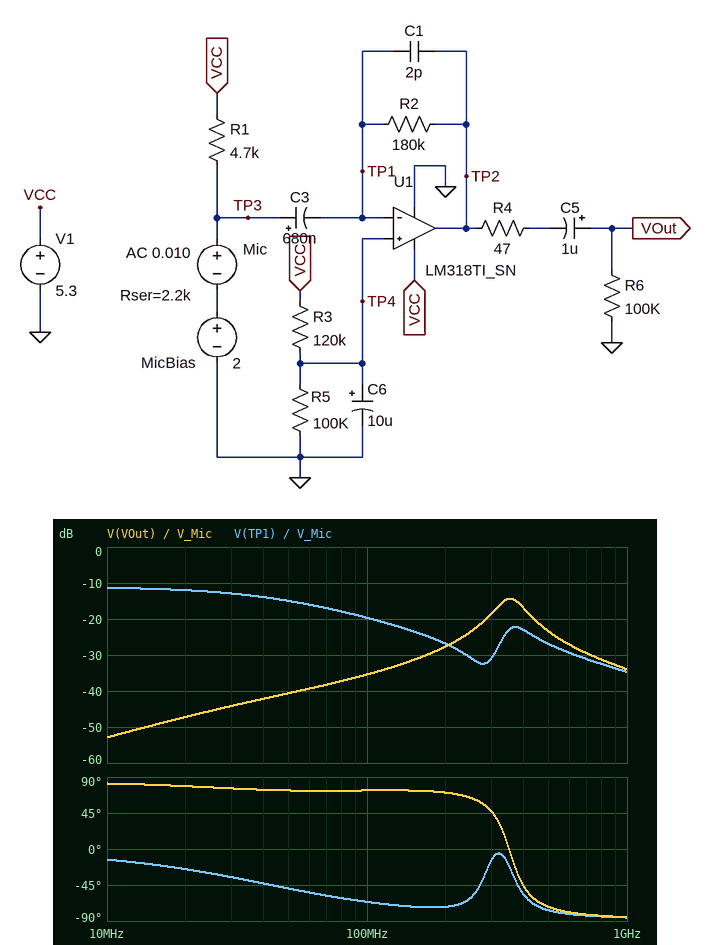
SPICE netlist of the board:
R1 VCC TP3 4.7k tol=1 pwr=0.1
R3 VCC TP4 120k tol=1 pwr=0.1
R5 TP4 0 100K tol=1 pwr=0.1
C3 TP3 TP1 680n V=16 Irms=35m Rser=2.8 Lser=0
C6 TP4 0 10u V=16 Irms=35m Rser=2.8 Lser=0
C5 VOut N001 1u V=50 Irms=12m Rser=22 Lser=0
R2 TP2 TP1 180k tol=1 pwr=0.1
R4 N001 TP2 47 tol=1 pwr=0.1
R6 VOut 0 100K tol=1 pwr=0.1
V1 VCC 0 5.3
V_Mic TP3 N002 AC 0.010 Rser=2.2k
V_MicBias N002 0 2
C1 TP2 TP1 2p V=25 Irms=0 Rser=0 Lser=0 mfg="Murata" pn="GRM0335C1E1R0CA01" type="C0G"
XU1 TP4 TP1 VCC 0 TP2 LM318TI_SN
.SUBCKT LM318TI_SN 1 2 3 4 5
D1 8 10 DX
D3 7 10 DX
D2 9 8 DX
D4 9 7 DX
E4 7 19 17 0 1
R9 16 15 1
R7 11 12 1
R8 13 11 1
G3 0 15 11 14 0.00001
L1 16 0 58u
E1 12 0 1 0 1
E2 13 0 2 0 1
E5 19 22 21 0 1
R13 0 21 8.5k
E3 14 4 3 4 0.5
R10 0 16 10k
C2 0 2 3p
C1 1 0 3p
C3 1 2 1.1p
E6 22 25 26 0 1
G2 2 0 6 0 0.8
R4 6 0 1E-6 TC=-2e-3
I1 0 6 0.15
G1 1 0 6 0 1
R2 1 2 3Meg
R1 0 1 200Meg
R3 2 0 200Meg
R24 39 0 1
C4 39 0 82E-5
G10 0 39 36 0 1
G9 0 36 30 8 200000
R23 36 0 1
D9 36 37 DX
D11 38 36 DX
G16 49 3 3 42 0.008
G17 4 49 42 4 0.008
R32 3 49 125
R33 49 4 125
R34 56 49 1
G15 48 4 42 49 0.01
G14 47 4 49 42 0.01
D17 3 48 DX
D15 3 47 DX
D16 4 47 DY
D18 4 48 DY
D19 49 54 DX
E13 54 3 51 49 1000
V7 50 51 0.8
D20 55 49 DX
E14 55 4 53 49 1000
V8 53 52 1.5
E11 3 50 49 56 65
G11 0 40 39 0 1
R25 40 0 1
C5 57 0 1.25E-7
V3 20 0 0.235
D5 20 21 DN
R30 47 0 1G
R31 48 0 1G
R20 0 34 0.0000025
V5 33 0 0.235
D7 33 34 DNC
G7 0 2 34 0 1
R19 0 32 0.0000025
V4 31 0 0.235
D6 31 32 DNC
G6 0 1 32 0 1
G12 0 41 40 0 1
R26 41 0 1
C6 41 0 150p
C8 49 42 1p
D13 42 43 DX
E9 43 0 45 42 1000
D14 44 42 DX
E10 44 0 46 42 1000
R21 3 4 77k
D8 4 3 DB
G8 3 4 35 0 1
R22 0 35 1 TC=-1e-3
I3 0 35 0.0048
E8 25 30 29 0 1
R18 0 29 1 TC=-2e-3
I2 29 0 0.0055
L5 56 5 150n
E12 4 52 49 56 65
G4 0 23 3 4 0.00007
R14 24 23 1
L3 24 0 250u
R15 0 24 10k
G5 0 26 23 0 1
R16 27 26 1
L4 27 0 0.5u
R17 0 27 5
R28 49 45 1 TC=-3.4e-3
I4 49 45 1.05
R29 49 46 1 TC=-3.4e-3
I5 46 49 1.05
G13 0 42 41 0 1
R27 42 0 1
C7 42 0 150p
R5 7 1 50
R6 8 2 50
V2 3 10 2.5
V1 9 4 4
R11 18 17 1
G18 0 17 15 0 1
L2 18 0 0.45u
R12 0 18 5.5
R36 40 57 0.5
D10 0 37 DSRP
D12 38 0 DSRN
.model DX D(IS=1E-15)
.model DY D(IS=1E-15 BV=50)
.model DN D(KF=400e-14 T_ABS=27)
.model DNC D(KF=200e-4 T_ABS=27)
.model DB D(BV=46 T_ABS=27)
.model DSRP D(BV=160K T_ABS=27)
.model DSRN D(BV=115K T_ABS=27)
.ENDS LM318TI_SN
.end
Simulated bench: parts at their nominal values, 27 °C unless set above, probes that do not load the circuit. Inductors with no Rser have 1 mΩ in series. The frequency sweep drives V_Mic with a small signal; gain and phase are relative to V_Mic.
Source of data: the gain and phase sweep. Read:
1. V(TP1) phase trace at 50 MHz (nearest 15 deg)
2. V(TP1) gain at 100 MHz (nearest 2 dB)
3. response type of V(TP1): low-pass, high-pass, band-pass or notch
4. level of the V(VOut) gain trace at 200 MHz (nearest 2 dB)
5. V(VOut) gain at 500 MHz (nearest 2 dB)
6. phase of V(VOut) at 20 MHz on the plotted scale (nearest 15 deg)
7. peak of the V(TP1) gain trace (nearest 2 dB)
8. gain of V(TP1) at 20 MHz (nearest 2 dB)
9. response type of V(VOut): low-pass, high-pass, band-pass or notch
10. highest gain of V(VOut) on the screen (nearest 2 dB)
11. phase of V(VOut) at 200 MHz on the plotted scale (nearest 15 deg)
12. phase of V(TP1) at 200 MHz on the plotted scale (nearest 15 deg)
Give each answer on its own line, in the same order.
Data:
-45 deg
-20 dB
low-pass
-28 dB
-24 dB
75 deg
-12 dB
-12 dB
band-pass
-14 dB
75 deg
-75 deg
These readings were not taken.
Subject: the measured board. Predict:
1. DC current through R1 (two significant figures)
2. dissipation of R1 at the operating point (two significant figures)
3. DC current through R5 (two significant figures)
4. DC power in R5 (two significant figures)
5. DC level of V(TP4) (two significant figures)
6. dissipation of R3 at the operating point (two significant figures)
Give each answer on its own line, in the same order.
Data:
480 µA
1.1 mW
34 µA
110 µW
3.4 V
31 µW
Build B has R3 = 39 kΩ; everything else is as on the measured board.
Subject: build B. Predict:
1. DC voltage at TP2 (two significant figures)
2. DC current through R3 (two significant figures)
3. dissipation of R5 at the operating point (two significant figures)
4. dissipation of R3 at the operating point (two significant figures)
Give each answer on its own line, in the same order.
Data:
4.5 V
48 µA
120 µW
91 µW
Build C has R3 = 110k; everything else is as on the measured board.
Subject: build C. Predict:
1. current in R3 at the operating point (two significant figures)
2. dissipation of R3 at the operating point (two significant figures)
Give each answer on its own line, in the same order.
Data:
17 µA
33 µW
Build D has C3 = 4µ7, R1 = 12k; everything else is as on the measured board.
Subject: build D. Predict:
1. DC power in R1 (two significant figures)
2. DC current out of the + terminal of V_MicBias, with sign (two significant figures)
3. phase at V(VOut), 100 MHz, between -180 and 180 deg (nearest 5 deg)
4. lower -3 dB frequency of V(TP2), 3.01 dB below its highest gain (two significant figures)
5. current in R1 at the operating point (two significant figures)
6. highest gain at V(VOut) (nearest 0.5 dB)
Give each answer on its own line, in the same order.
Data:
650 µW
-230 µA
70 deg
310 MHz
230 µA
-14.0 dB
